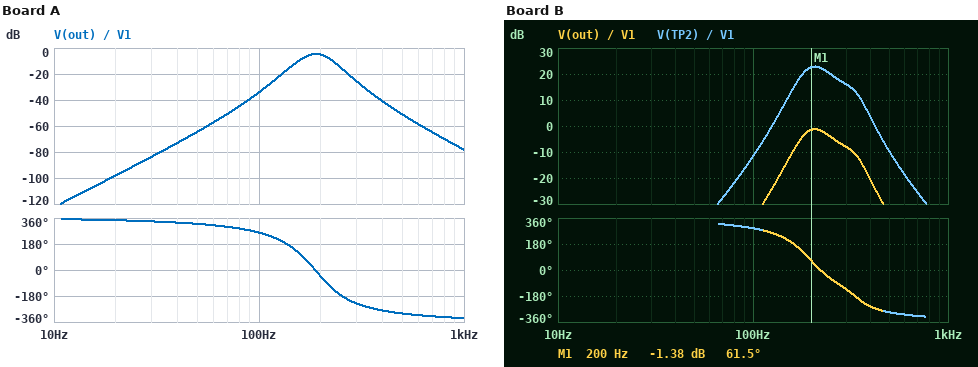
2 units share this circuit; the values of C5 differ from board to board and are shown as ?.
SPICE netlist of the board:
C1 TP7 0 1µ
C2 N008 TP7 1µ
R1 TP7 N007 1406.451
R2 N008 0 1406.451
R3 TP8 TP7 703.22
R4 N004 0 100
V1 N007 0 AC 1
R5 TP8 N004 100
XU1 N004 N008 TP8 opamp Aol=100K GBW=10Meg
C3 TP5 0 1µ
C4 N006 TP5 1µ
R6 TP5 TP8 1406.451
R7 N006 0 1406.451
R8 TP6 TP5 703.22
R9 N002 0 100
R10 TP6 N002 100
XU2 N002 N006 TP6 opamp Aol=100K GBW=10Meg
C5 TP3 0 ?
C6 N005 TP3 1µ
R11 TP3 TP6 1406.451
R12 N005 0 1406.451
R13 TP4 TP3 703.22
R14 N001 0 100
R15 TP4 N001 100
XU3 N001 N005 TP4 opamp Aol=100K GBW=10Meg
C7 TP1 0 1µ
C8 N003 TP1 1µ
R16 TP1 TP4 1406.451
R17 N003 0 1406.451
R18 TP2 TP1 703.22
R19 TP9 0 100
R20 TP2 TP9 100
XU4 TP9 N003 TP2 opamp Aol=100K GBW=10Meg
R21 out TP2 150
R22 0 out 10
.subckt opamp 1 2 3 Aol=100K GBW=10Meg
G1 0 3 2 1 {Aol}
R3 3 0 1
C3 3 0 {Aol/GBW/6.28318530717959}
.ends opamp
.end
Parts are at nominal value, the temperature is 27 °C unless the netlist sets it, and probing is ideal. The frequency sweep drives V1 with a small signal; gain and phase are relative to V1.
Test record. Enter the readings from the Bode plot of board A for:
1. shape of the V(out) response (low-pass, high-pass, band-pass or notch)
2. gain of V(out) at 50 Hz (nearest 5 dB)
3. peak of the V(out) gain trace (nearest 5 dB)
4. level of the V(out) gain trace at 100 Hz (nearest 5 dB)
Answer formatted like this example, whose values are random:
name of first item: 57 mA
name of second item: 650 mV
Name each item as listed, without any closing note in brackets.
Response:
shape of the V(out) response: band-pass
gain of V(out) at 50 Hz: -65 dB
peak of the V(out) gain trace: -5 dB
level of the V(out) gain trace at 100 Hz: -35 dB
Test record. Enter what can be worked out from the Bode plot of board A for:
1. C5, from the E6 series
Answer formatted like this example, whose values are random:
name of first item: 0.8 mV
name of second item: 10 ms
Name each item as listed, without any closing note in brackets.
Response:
C5, from the E6 series: 1.5 µF
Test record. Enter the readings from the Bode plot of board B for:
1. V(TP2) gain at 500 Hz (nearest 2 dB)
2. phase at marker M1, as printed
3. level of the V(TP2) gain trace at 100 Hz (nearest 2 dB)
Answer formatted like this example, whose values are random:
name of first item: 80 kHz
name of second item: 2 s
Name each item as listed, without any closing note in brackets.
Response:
V(TP2) gain at 500 Hz: -10 dB
phase at marker M1, as printed: 61.5 deg
level of the V(TP2) gain trace at 100 Hz: -12 dB
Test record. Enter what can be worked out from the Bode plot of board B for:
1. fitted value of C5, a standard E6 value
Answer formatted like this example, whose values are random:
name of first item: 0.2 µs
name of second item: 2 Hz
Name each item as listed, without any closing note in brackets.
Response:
fitted value of C5, a standard E6 value: 330 nF
